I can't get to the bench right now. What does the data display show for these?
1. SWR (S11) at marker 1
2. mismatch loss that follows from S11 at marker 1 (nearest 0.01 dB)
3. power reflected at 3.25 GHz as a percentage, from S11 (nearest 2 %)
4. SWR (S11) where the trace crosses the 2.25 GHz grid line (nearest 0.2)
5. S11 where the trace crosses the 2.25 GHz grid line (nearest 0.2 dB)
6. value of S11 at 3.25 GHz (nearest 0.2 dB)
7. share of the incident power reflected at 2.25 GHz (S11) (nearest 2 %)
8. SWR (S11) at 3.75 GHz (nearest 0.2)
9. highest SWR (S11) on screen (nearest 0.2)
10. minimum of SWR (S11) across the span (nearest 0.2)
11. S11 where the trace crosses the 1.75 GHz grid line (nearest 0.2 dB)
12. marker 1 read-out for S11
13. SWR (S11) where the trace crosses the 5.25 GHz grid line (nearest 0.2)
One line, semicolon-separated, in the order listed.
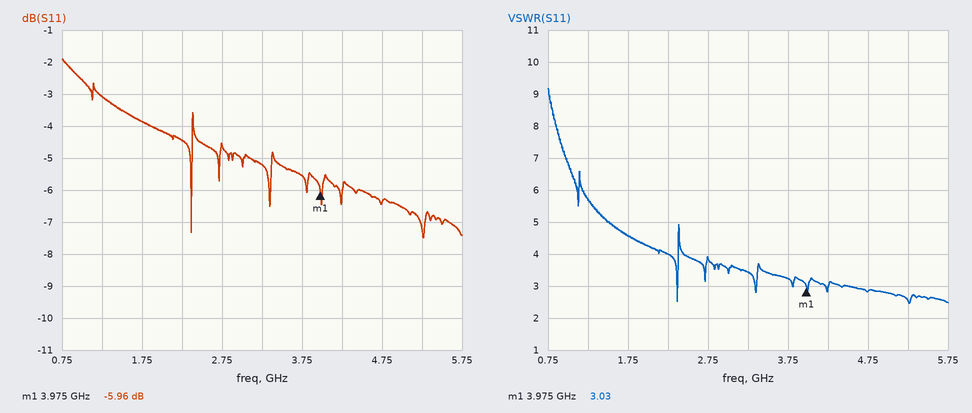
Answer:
3.03; 1.27 dB; 30 %; 4.0; -4.4 dB; -5.2 dB; 36 %; 3.2; 9.2; 2.4; -3.8 dB; -5.96 dB; 2.6
